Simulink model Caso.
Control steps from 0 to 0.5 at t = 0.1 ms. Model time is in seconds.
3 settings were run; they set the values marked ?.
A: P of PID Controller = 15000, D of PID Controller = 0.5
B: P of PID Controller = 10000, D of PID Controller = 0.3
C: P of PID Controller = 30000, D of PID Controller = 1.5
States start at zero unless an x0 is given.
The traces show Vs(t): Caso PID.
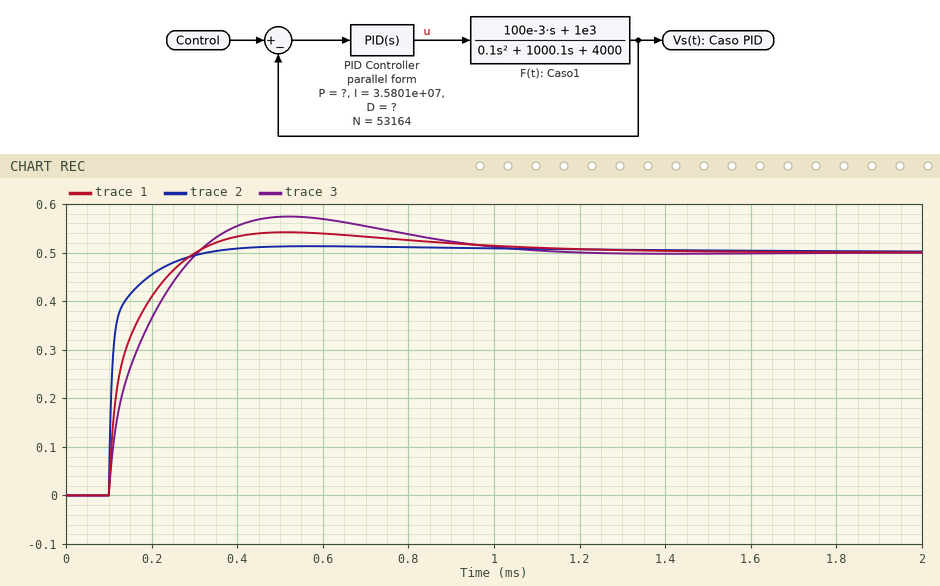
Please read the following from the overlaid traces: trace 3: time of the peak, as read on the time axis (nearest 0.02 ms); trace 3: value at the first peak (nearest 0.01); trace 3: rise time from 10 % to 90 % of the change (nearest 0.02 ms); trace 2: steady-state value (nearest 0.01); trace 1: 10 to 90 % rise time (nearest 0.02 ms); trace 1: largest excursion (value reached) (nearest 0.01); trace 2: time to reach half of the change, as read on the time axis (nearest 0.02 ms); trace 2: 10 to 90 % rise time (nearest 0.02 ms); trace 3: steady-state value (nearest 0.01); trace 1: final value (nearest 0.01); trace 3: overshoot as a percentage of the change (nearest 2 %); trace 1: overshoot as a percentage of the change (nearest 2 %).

0.52 ms
0.57
0.16 ms
0.50
0.14 ms
0.54
0.10 ms
0.10 ms
0.50
0.50
14 %
8 %
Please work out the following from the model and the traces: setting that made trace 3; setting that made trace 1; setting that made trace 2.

B
A
C
